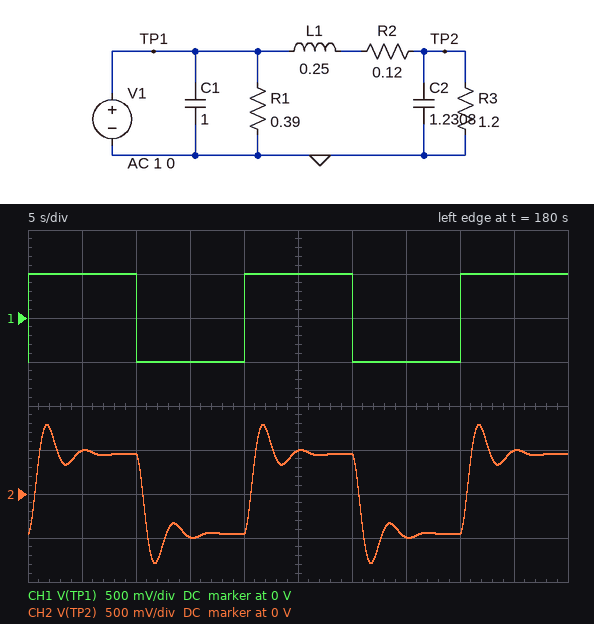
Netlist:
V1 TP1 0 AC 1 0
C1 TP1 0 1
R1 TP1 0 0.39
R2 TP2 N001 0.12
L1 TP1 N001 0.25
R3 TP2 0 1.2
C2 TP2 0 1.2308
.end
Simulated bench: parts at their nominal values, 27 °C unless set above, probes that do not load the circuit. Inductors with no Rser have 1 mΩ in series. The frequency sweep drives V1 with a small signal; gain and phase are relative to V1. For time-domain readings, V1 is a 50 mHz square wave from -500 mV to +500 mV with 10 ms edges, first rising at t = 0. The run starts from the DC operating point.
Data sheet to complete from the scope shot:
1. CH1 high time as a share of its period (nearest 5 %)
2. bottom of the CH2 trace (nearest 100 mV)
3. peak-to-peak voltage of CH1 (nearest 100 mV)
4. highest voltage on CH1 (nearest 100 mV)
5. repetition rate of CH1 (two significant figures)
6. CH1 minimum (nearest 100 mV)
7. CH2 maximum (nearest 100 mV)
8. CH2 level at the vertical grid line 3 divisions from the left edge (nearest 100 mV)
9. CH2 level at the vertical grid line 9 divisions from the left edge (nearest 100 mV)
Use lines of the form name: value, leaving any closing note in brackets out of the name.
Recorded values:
CH1 high time as a share of its period: 50 %
bottom of the CH2 trace: -800 mV
peak-to-peak voltage of CH1: 1.0 V
highest voltage on CH1: 500 mV
repetition rate of CH1: 50 mHz
CH1 minimum: -500 mV
CH2 maximum: 800 mV
CH2 level at the vertical grid line 3 divisions from the left edge: -500 mV
CH2 level at the vertical grid line 9 divisions from the left edge: 500 mV
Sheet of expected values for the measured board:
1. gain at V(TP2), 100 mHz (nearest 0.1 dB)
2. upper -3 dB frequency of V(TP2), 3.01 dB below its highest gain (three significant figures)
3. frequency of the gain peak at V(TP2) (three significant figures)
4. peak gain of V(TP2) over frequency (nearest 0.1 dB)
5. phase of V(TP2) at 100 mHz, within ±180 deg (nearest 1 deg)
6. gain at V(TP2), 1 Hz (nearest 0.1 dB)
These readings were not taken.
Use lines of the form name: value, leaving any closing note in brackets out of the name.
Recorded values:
gain at V(TP2), 100 mHz: 0 dB
upper -3 dB frequency of V(TP2), 3.01 dB below its highest gain: 356 mHz
frequency of the gain peak at V(TP2): 271 mHz
peak gain of V(TP2) over frequency: 3.8 dB
phase of V(TP2) at 100 mHz, within ±180 deg: -13 deg
gain at V(TP2), 1 Hz: -21.0 dB
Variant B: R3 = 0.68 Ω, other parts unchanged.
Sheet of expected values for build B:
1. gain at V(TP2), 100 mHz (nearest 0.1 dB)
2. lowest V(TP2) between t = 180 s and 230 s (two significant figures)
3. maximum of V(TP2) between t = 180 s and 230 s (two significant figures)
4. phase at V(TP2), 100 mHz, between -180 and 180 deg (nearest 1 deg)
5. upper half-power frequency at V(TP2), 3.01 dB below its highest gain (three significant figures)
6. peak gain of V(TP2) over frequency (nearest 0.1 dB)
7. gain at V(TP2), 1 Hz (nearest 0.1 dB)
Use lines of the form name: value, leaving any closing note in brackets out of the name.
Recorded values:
gain at V(TP2), 100 mHz: -0.9 dB
lowest V(TP2) between t = 180 s and 230 s: -620 mV
maximum of V(TP2) between t = 180 s and 230 s: 620 mV
phase at V(TP2), 100 mHz, between -180 and 180 deg: -17 deg
upper half-power frequency at V(TP2), 3.01 dB below its highest gain: 369 mHz
peak gain of V(TP2) over frequency: 0.8 dB
gain at V(TP2), 1 Hz: -21.2 dB
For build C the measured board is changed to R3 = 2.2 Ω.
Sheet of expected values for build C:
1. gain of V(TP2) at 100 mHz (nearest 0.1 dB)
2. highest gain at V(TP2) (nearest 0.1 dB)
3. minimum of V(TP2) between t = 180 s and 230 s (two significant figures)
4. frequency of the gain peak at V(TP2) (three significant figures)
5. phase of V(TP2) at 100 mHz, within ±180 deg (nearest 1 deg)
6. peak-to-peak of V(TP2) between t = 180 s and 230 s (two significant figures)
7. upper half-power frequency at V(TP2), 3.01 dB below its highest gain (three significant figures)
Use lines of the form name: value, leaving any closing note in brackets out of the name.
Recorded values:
gain of V(TP2) at 100 mHz: 0.5 dB
highest gain at V(TP2): 6.5 dB
minimum of V(TP2) between t = 180 s and 230 s: -920 mV
frequency of the gain peak at V(TP2): 279 mHz
phase of V(TP2) at 100 mHz, within ±180 deg: -10 deg
peak-to-peak of V(TP2) between t = 180 s and 230 s: 1.8 V
upper half-power frequency at V(TP2), 3.01 dB below its highest gain: 341 mHz
